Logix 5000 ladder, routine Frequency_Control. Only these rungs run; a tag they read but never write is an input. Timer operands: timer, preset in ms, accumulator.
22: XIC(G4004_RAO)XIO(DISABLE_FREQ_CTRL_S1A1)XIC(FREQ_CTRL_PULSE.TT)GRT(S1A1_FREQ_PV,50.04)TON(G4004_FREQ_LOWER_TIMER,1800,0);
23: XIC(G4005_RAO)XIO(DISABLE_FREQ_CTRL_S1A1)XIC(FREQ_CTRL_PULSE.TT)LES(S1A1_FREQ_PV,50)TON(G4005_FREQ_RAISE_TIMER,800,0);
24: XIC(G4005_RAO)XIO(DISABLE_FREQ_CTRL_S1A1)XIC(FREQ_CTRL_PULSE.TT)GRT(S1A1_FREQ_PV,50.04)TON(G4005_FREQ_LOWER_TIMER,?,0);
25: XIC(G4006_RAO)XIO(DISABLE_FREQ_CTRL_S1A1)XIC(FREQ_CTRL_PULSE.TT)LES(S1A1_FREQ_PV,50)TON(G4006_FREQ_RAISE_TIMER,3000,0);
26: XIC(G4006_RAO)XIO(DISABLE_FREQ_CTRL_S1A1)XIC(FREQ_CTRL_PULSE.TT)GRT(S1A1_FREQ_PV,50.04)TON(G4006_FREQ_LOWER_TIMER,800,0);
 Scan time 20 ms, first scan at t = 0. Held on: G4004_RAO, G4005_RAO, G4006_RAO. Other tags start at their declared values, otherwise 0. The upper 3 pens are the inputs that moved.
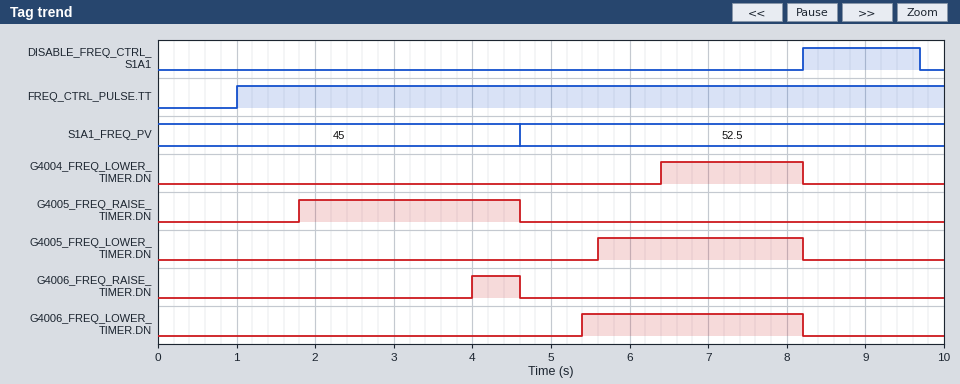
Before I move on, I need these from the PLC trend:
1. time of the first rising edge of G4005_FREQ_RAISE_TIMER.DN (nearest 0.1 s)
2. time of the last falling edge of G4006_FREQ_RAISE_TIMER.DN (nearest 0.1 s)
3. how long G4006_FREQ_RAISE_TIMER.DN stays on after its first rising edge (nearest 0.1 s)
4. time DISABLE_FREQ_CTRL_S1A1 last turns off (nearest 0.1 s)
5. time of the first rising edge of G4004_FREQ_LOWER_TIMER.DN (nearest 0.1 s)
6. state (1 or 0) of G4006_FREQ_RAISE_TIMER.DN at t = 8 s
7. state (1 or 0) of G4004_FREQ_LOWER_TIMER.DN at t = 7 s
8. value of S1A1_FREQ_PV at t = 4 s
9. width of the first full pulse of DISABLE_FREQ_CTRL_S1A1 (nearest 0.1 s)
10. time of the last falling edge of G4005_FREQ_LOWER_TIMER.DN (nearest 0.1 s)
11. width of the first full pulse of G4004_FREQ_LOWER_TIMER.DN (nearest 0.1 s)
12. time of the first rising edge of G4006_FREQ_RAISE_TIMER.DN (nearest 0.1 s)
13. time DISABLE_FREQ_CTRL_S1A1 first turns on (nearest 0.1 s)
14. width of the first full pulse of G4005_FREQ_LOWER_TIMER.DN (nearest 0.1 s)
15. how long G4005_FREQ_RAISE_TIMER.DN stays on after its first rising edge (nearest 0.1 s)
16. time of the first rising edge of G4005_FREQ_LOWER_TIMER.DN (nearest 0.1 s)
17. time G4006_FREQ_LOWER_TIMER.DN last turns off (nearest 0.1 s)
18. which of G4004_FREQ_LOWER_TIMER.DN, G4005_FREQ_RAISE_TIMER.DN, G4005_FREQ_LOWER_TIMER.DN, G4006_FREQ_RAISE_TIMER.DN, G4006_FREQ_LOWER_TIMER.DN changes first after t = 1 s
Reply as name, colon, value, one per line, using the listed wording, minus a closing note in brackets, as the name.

time of the first rising edge of G4005_FREQ_RAISE_TIMER.DN: 1.8 s
time of the last falling edge of G4006_FREQ_RAISE_TIMER.DN: 4.6 s
how long G4006_FREQ_RAISE_TIMER.DN stays on after its first rising edge: 0.6 s
time DISABLE_FREQ_CTRL_S1A1 last turns off: 9.7 s
time of the first rising edge of G4004_FREQ_LOWER_TIMER.DN: 6.4 s
state (1 or 0) of G4006_FREQ_RAISE_TIMER.DN at t = 8 s: 0
state (1 or 0) of G4004_FREQ_LOWER_TIMER.DN at t = 7 s: 1
value of S1A1_FREQ_PV at t = 4 s: 45
width of the first full pulse of DISABLE_FREQ_CTRL_S1A1: 1.5 s
time of the last falling edge of G4005_FREQ_LOWER_TIMER.DN: 8.2 s
width of the first full pulse of G4004_FREQ_LOWER_TIMER.DN: 1.8 s
time of the first rising edge of G4006_FREQ_RAISE_TIMER.DN: 4.0 s
time DISABLE_FREQ_CTRL_S1A1 first turns on: 8.2 s
width of the first full pulse of G4005_FREQ_LOWER_TIMER.DN: 2.6 s
how long G4005_FREQ_RAISE_TIMER.DN stays on after its first rising edge: 2.8 s
time of the first rising edge of G4005_FREQ_LOWER_TIMER.DN: 5.6 s
time G4006_FREQ_LOWER_TIMER.DN last turns off: 8.2 s
which of G4004_FREQ_LOWER_TIMER.DN, G4005_FREQ_RAISE_TIMER.DN, G4005_FREQ_LOWER_TIMER.DN, G4006_FREQ_RAISE_TIMER.DN, G4006_FREQ_LOWER_TIMER.DN changes first after t = 1 s: G4005_FREQ_RAISE_TIMER.DN
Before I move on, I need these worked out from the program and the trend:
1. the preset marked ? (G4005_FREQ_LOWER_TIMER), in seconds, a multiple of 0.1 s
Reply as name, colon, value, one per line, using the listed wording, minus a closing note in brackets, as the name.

the preset marked ? (G4005_FREQ_LOWER_TIMER), in seconds, a multiple of 0.1 s: 1.0 s
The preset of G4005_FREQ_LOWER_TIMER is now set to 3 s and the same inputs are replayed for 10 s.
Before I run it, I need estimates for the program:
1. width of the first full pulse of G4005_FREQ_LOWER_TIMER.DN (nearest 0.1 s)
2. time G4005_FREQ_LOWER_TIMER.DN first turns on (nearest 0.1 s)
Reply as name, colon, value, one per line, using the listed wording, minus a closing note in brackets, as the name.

width of the first full pulse of G4005_FREQ_LOWER_TIMER.DN: 0.6 s
time G4005_FREQ_LOWER_TIMER.DN first turns on: 7.6 s
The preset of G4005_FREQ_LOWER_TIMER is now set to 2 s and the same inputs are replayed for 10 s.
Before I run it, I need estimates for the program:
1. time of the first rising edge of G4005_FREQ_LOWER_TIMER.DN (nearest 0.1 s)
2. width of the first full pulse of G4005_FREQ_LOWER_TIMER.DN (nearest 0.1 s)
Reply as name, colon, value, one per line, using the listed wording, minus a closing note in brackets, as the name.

time of the first rising edge of G4005_FREQ_LOWER_TIMER.DN: 6.6 s
width of the first full pulse of G4005_FREQ_LOWER_TIMER.DN: 1.6 s
